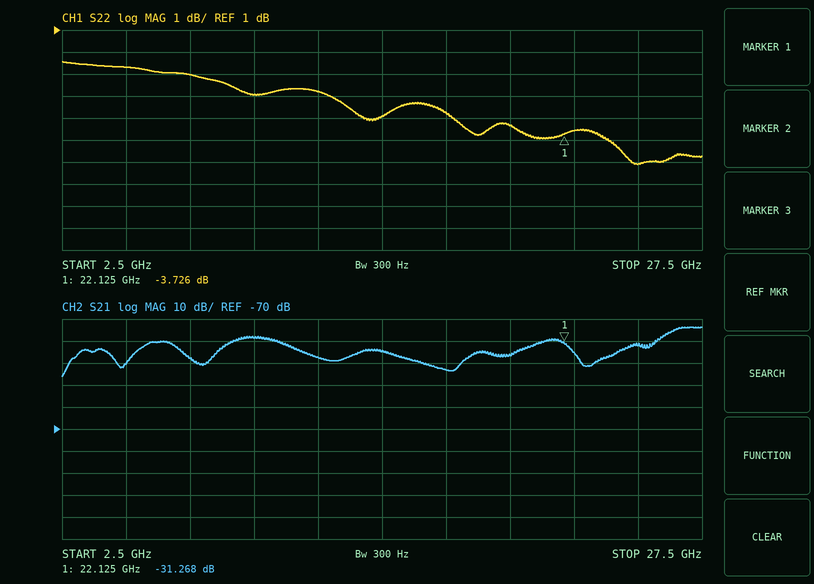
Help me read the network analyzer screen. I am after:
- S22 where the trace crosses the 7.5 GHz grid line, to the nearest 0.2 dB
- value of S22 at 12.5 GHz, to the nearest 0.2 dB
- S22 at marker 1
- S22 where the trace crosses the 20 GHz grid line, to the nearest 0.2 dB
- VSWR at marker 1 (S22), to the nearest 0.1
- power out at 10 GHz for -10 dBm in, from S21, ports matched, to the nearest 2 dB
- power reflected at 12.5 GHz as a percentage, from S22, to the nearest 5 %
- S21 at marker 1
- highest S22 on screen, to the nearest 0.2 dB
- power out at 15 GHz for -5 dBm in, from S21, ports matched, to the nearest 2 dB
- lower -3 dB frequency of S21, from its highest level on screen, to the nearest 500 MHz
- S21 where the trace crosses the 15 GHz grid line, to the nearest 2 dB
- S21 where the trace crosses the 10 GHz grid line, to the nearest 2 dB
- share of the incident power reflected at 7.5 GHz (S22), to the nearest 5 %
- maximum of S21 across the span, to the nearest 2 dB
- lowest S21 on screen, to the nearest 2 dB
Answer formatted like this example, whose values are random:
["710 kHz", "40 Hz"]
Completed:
["-1.0 dB", "-1.8 dB", "-3.726 dB", "-3.4 dB", "4.7", "-38 dBm", "65 %", "-31.268 dB", "-0.4 dB", "-40 dBm", "26.0 GHz", "-34 dB", "-28 dB", "80 %", "-24 dB", "-46 dB"]
